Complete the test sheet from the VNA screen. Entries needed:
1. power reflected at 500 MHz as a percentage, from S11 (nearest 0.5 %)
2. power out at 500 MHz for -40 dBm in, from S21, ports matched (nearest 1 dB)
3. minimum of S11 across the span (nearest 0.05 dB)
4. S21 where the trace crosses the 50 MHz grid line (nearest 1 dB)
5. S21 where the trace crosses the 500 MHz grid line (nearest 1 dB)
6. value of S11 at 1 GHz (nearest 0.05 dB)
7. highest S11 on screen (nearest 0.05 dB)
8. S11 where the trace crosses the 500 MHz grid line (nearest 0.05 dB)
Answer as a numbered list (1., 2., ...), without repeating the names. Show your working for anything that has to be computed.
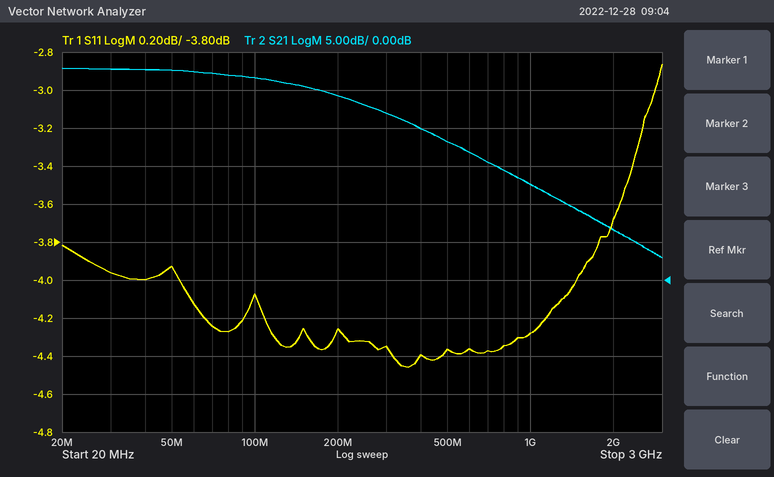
1. 10^(-4.35/10) ≈ 36.7 %, so 36.5 % to the nearest 0.5 %
2. -40 dBm + (18 dB) = -22 dBm
3. -4.45 dB
4. 28 dB
5. 18 dB
6. -4.30 dB
7. -2.85 dB
8. -4.35 dB
